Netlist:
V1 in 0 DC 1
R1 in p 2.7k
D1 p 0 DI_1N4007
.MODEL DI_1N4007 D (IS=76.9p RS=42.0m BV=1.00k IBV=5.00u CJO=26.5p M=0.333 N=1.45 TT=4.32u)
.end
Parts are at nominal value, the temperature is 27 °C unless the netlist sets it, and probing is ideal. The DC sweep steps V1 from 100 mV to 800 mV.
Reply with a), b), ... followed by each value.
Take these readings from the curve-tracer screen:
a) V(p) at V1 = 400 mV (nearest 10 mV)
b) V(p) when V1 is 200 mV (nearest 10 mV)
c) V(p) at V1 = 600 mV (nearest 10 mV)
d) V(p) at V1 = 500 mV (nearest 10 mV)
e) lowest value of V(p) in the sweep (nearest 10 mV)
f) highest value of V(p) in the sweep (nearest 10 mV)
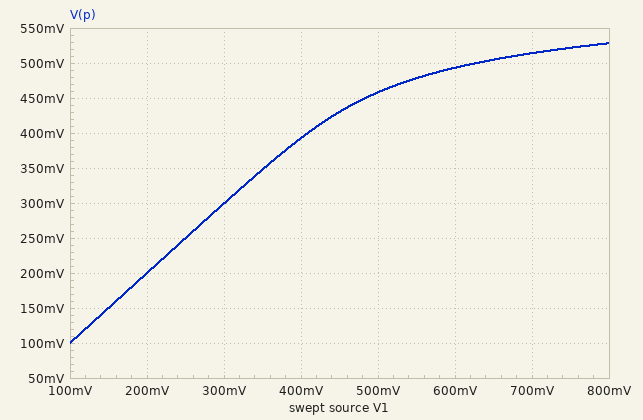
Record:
a) 390 mV
b) 200 mV
c) 490 mV
d) 460 mV
e) 100 mV
f) 530 mV
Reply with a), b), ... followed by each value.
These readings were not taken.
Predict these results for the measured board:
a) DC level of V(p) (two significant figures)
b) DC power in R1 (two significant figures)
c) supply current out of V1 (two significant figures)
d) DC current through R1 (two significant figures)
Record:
a) 550 mV
b) 76 µW
c) 170 µA
d) 170 µA
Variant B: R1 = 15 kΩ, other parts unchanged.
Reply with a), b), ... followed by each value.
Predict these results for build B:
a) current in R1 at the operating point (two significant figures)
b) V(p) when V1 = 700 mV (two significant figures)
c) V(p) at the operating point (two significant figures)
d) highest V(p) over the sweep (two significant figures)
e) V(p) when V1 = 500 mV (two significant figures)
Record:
a) 34 µA
b) 460 mV
c) 490 mV
d) 470 mV
e) 420 mV
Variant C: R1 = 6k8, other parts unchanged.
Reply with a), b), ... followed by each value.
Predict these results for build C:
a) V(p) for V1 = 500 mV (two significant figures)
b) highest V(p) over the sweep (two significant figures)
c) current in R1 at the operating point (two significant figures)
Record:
a) 440 mV
b) 500 mV
c) 71 µA
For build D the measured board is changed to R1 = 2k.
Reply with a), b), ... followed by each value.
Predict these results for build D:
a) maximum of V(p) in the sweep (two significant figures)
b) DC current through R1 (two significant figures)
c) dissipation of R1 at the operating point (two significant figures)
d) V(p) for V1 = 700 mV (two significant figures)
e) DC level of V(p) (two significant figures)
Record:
a) 540 mV
b) 220 µA
c) 98 µW
d) 520 mV
e) 560 mV
